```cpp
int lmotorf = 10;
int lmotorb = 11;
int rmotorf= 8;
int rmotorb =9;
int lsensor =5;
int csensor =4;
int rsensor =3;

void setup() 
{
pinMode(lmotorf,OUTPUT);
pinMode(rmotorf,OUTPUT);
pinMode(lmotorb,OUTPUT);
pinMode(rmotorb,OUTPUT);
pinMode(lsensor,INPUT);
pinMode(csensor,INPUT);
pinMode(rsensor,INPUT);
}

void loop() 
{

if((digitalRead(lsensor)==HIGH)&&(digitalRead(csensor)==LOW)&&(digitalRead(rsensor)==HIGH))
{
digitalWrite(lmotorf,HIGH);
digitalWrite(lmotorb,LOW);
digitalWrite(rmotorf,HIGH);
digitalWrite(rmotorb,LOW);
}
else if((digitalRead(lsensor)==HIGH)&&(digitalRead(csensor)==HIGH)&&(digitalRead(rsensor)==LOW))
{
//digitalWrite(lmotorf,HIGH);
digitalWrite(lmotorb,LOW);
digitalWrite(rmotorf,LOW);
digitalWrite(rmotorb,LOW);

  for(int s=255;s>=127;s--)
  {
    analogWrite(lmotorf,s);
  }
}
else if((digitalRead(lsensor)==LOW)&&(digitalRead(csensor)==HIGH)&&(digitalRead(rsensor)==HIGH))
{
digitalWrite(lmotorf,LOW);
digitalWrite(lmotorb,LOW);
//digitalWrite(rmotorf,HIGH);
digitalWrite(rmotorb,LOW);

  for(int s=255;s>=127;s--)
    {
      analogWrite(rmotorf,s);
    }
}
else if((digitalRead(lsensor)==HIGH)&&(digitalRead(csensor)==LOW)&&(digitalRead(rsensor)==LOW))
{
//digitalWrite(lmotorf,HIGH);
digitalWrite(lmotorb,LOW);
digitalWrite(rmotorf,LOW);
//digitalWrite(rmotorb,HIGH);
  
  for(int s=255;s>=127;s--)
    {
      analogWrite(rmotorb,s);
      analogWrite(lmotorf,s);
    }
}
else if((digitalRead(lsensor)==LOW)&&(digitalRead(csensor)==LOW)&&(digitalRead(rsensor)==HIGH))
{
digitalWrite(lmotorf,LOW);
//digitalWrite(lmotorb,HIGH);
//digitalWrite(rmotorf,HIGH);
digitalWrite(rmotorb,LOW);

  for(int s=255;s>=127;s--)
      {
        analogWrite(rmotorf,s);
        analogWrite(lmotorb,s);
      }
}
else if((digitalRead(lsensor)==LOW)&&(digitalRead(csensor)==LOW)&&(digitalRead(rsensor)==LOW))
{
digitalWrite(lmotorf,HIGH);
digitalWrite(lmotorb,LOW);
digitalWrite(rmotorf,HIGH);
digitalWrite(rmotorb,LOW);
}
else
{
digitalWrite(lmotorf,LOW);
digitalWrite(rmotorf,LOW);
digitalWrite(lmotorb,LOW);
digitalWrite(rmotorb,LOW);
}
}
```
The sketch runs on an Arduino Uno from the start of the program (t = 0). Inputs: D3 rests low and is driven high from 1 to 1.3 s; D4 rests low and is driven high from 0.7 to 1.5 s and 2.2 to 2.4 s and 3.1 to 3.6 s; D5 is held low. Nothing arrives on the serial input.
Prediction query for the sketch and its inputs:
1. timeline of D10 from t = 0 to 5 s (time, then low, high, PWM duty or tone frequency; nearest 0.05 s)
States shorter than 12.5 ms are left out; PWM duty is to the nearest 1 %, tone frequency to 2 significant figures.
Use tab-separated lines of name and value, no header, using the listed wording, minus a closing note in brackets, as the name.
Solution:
timeline of D10 from t = 0 to 5 s	0 s high; 0.7 s low; 1.5 s high; 2.2 s low; 2.4 s high; 3.1 s low; 3.6 s high
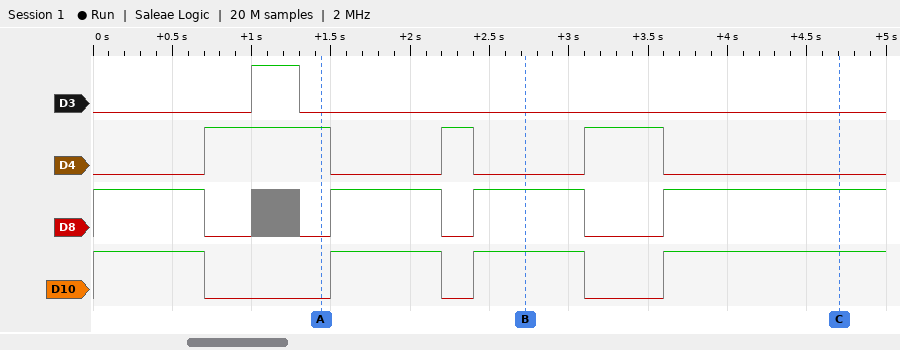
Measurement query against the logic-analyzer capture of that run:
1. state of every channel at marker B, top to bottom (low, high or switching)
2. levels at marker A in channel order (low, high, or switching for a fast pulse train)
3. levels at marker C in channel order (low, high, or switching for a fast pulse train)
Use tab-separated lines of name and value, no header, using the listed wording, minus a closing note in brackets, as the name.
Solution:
state of every channel at marker B, top to bottom	D3 low, D4 low, D8 high, D10 high
levels at marker A in channel order	D3 low, D4 high, D8 low, D10 low
levels at marker C in channel order	D3 low, D4 low, D8 high, D10 high
